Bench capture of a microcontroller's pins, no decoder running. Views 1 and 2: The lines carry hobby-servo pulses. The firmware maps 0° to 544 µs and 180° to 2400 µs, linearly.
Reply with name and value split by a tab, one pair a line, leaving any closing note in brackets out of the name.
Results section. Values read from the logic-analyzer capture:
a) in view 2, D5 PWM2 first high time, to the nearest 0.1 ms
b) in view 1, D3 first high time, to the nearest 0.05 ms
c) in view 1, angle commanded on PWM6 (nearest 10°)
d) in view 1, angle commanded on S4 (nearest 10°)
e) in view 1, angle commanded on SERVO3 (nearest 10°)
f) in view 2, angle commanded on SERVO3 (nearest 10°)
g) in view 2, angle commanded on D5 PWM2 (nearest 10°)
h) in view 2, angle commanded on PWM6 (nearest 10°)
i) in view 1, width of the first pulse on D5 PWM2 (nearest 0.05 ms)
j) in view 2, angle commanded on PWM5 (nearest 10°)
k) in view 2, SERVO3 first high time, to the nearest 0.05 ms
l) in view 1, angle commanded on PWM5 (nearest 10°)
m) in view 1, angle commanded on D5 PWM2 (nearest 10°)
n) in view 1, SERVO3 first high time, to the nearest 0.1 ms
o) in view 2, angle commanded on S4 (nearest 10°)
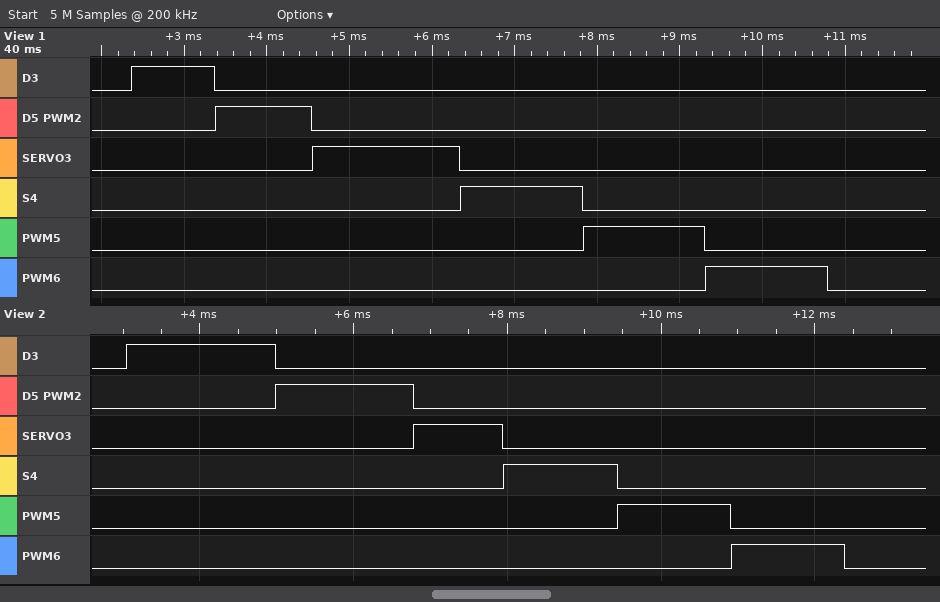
in view 2, D5 PWM2 first high time, to the nearest 0.1 ms	1.8 ms
in view 1, D3 first high time, to the nearest 0.05 ms	1.00 ms
in view 1, angle commanded on PWM6	90°
in view 1, angle commanded on S4	90°
in view 1, angle commanded on SERVO3	120°
in view 2, angle commanded on SERVO3	60°
in view 2, angle commanded on D5 PWM2	120°
in view 2, angle commanded on PWM6	90°
in view 1, width of the first pulse on D5 PWM2	1.15 ms
in view 2, angle commanded on PWM5	90°
in view 2, SERVO3 first high time, to the nearest 0.05 ms	1.15 ms
in view 1, angle commanded on PWM5	90°
in view 1, angle commanded on D5 PWM2	60°
in view 1, SERVO3 first high time, to the nearest 0.1 ms	1.8 ms
in view 2, angle commanded on S4	90°
